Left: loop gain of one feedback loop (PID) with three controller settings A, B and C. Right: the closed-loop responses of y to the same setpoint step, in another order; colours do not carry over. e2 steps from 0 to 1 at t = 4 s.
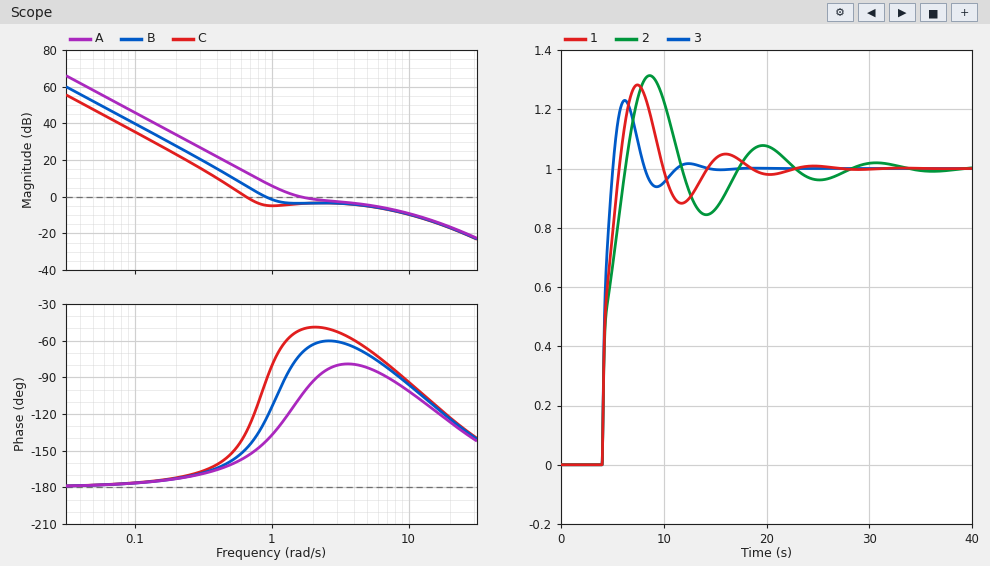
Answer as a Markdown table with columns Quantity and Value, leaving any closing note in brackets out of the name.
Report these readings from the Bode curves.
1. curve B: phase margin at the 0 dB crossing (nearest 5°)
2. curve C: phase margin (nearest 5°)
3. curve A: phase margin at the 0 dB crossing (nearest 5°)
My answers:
| Quantity | Value |
|---|---|
| curve B: phase margin at the 0 dB crossing | 55° |
| curve C: phase margin | 45° |
| curve A: phase margin at the 0 dB crossing | 75° |
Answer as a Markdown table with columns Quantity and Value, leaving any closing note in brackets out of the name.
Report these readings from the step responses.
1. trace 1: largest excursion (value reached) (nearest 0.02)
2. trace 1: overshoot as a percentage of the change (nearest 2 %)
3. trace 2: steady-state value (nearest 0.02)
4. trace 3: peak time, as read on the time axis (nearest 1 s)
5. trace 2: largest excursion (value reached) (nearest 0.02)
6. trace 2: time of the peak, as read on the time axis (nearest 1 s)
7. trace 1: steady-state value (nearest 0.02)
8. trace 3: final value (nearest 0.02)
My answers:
| Quantity | Value |
|---|---|
| trace 1: largest excursion (value reached) | 1.28 |
| trace 1: overshoot as a percentage of the change | 28 % |
| trace 2: steady-state value | 1.00 |
| trace 3: peak time, as read on the time axis | 6 s |
| trace 2: largest excursion (value reached) | 1.32 |
| trace 2: time of the peak, as read on the time axis | 9 s |
| trace 1: steady-state value | 1.00 |
| trace 3: final value | 1.00 |
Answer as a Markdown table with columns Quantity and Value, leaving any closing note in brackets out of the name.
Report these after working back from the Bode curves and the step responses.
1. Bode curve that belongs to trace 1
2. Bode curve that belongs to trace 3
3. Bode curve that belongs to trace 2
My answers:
| Quantity | Value |
|---|---|
| Bode curve that belongs to trace 1 | B |
| Bode curve that belongs to trace 3 | A |
| Bode curve that belongs to trace 2 | C |
